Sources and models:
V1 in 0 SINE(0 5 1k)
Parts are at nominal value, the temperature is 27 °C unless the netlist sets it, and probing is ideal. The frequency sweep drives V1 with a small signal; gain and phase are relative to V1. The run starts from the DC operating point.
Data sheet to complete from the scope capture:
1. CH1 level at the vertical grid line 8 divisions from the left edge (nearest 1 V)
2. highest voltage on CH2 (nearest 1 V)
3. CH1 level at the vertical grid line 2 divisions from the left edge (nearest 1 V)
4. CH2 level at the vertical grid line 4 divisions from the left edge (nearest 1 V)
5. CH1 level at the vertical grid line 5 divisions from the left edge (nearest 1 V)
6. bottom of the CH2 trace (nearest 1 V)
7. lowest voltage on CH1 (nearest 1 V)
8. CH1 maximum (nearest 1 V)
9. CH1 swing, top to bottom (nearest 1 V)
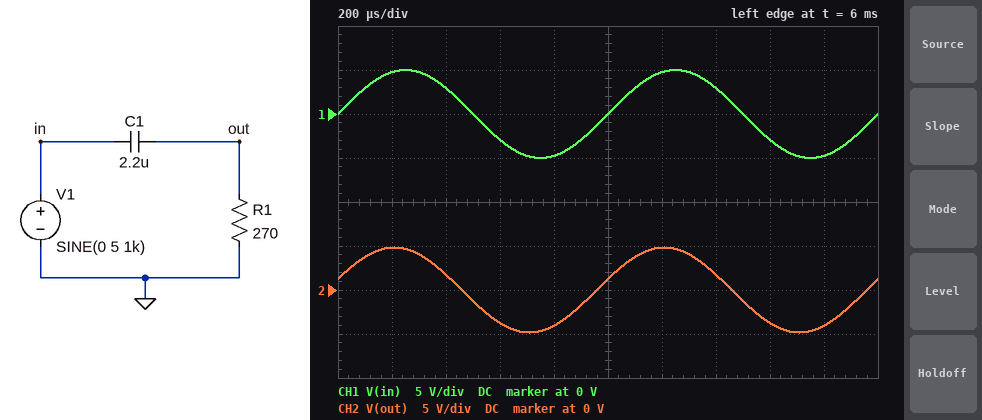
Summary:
-3 V
5 V
3 V
-4 V
0 V
-5 V
-5 V
5 V
10 V
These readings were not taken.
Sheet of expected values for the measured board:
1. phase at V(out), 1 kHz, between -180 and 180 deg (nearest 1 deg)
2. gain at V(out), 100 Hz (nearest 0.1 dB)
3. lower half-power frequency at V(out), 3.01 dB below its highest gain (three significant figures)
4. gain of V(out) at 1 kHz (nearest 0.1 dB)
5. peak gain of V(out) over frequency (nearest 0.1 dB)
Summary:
15 deg
-9.1 dB
268 Hz
-0.3 dB
0 dB
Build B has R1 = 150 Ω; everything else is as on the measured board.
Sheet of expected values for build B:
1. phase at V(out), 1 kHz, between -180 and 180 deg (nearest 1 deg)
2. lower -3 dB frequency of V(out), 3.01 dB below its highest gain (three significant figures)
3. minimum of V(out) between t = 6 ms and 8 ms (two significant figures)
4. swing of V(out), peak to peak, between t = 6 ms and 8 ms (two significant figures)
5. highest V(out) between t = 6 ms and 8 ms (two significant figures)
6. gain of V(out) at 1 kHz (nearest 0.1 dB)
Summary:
26 deg
482 Hz
-4.5 V
9.0 V
4.5 V
-0.9 dB
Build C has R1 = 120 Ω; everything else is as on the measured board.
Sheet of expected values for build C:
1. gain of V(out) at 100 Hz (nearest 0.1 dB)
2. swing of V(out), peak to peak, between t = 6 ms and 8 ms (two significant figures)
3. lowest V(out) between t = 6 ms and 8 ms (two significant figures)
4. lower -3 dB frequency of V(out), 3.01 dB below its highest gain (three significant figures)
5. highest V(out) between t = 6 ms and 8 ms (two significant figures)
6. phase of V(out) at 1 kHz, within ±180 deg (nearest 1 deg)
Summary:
-15.7 dB
8.6 V
-4.3 V
603 Hz
4.3 V
31 deg
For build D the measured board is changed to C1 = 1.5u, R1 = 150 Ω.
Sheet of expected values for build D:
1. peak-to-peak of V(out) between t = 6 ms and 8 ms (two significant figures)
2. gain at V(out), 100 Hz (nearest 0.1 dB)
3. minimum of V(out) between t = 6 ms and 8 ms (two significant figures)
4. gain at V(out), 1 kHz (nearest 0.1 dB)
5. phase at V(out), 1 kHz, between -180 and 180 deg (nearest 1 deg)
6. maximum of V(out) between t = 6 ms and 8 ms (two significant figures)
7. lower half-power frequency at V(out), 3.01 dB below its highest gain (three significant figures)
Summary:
8.2 V
-17.1 dB
-4.1 V
-1.8 dB
35 deg
4.1 V
707 Hz
